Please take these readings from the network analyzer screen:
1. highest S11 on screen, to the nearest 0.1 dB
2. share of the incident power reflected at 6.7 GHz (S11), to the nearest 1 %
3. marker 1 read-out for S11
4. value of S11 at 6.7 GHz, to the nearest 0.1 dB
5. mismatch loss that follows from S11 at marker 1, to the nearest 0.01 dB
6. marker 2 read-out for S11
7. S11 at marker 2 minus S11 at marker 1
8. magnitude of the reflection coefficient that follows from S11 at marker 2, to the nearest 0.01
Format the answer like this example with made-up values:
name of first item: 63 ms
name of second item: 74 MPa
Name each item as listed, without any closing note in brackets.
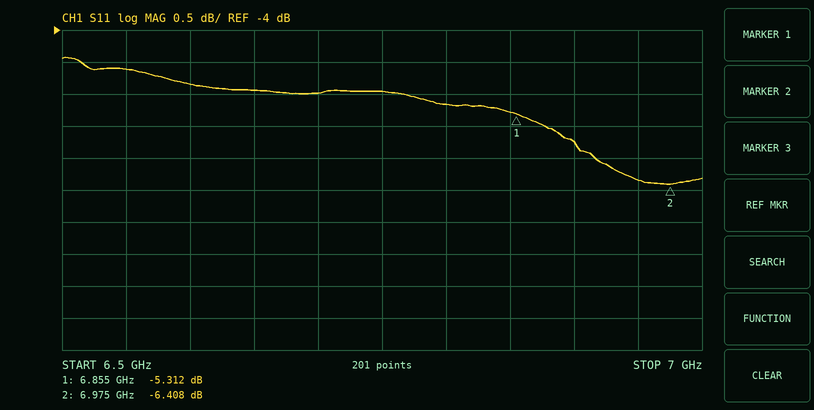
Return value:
highest S11 on screen, to the nearest 0.1 dB: -4.4 dB
share of the incident power reflected at 6.7 GHz (S11), to the nearest 1 %: 32 %
marker 1 read-out for S11: -5.312 dB
value of S11 at 6.7 GHz, to the nearest 0.1 dB: -5.0 dB
mismatch loss that follows from S11 at marker 1, to the nearest 0.01 dB: 1.51 dB
marker 2 read-out for S11: -6.408 dB
S11 at marker 2 minus S11 at marker 1: -1.096 dB
magnitude of the reflection coefficient that follows from S11 at marker 2, to the nearest 0.01: 0.48
